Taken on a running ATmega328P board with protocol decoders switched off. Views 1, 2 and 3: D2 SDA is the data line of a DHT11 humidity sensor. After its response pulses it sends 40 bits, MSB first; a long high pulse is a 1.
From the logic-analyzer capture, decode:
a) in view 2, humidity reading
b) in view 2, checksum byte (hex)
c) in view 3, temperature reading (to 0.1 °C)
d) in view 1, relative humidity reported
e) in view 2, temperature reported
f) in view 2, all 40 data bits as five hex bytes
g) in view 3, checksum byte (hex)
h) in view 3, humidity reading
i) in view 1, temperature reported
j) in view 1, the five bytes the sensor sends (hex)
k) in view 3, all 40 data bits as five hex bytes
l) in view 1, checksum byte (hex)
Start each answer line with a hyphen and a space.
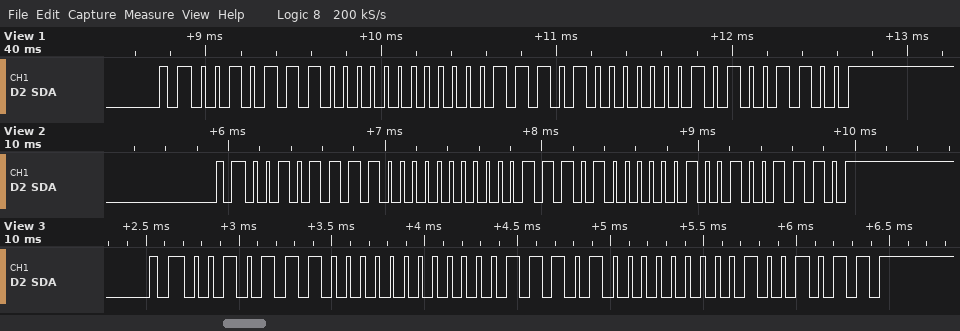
- 47 %
- 0x4E
- 29.0 °C
- 46 %
- 29.2 °C
- 2F 00 1D 02 4E
- 0x4B
- 46 %
- 29.1 °C
- 2E 00 1D 01 4C
- 2E 00 1D 00 4B
- 0x4C
